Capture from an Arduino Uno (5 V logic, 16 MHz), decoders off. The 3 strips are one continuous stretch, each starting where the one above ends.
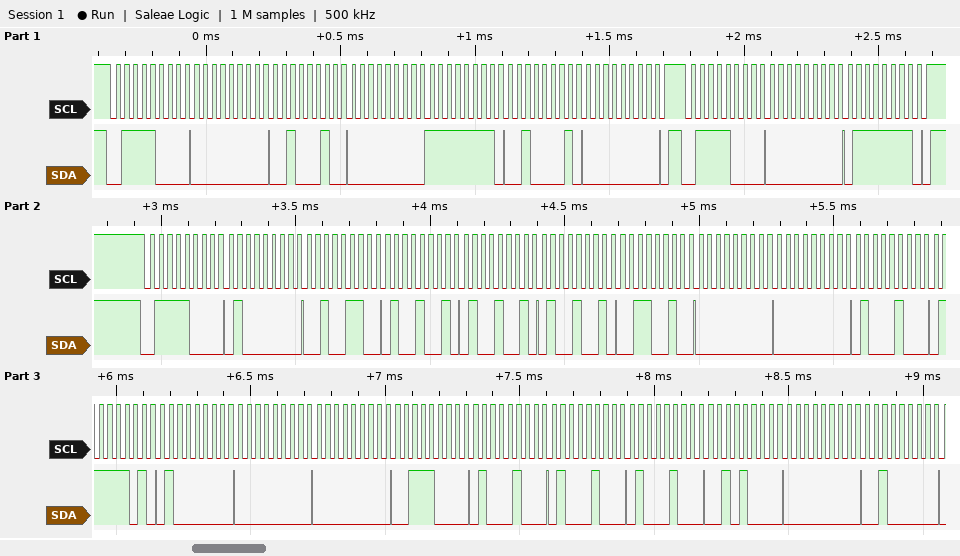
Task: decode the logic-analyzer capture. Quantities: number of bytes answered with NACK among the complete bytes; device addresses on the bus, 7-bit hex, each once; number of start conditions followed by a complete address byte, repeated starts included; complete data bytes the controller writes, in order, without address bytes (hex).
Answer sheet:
0
0x3C
3
00 22 00 FF 21 00 00 7F 40 26 49 49 49 32 00 00 44 7D 40 00 00 38 44 44 44 28 00 20
